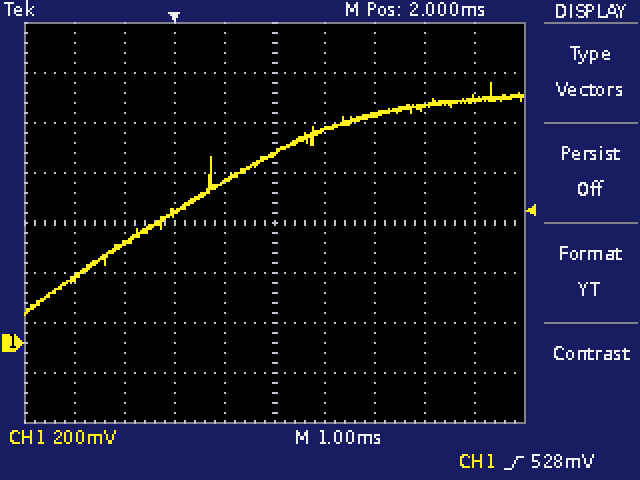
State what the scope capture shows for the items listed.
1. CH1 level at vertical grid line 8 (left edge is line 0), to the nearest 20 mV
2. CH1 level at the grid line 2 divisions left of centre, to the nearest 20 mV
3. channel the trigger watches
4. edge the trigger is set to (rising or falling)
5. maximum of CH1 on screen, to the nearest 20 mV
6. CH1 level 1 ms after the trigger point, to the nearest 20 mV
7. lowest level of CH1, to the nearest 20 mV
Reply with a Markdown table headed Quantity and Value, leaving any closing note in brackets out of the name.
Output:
| Quantity | Value |
|---|---|
| CH1 level at vertical grid line 8 (left edge is line 0), to the nearest 20 mV | 940 mV |
| CH1 level at the grid line 2 divisions left of centre, to the nearest 20 mV | 520 mV |
| channel the trigger watches | CH1 |
| edge the trigger is set to | rising |
| maximum of CH1 on screen, to the nearest 20 mV | 1.04 V |
| CH1 level 1 ms after the trigger point, to the nearest 20 mV | 640 mV |
| lowest level of CH1, to the nearest 20 mV | 120 mV |
